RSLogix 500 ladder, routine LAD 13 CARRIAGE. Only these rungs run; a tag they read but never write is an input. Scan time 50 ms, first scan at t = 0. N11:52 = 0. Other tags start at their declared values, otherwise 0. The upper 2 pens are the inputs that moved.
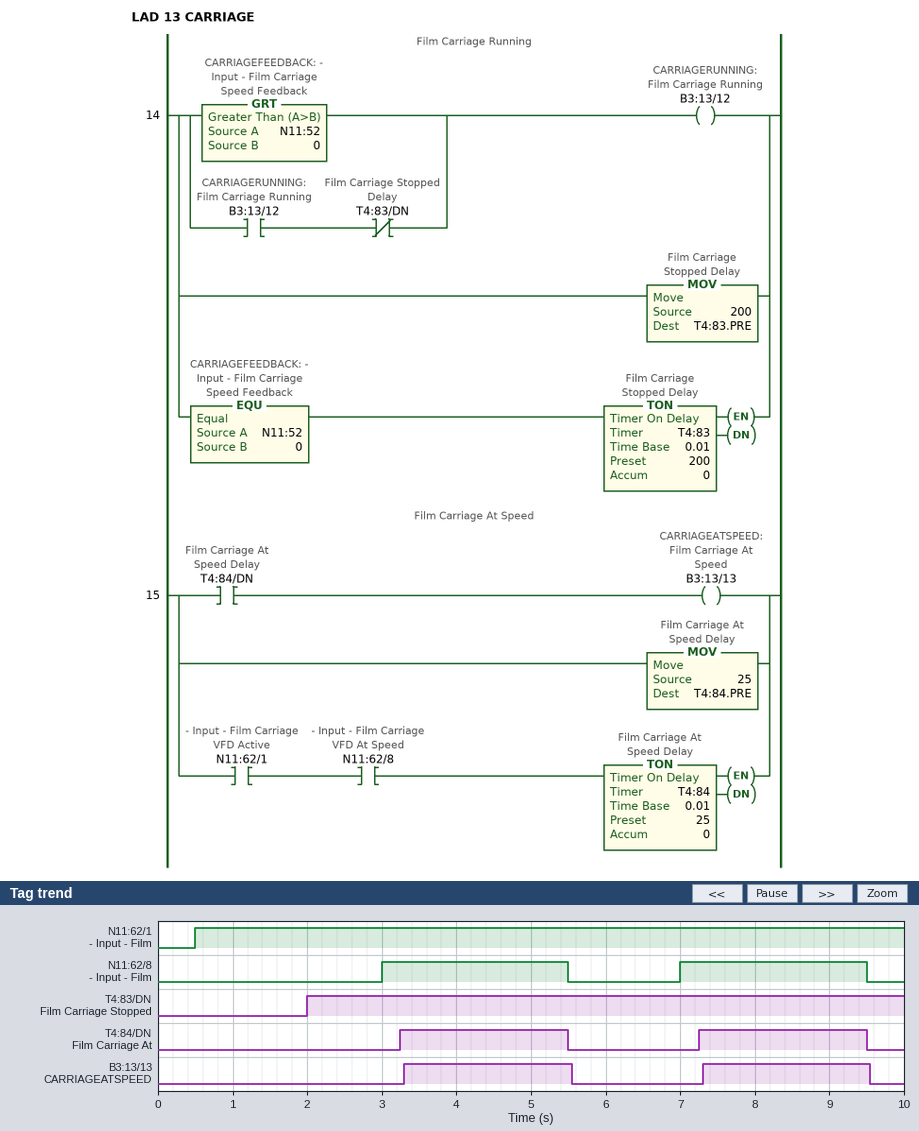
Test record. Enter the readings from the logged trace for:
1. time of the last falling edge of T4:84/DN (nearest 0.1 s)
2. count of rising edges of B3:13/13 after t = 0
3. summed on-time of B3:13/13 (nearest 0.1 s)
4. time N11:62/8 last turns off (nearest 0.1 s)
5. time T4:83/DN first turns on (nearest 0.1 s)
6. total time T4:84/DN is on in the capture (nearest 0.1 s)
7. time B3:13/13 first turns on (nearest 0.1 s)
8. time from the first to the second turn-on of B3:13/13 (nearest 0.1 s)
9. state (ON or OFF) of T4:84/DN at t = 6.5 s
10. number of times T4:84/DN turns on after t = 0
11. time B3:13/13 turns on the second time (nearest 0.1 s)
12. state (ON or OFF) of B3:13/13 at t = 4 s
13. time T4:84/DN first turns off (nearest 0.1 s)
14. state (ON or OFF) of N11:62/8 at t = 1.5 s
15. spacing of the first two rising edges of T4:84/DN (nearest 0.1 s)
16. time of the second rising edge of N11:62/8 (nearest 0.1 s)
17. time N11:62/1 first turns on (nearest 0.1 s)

9.5 s
2
4.5 s
9.5 s
2.0 s
4.5 s
3.3 s
4.0 s
OFF
2
7.3 s
ON
5.5 s
OFF
4.0 s
7.0 s
0.5 s
